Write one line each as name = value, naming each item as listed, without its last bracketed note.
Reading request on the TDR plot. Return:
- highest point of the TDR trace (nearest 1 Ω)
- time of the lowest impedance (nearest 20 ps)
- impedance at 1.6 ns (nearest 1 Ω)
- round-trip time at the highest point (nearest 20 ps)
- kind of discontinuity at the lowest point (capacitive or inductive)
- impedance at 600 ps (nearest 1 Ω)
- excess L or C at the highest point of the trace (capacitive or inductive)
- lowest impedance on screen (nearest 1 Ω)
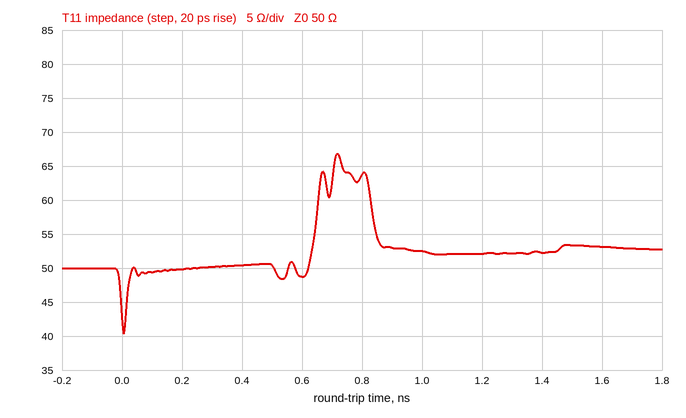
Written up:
highest point of the TDR trace = 67 Ω
time of the lowest impedance = 0 ps
impedance at 1.6 ns = 53 Ω
round-trip time at the highest point = 720 ps
kind of discontinuity at the lowest point = capacitive
impedance at 600 ps = 49 Ω
excess L or C at the highest point of the trace = inductive
lowest impedance on screen = 40 Ω
